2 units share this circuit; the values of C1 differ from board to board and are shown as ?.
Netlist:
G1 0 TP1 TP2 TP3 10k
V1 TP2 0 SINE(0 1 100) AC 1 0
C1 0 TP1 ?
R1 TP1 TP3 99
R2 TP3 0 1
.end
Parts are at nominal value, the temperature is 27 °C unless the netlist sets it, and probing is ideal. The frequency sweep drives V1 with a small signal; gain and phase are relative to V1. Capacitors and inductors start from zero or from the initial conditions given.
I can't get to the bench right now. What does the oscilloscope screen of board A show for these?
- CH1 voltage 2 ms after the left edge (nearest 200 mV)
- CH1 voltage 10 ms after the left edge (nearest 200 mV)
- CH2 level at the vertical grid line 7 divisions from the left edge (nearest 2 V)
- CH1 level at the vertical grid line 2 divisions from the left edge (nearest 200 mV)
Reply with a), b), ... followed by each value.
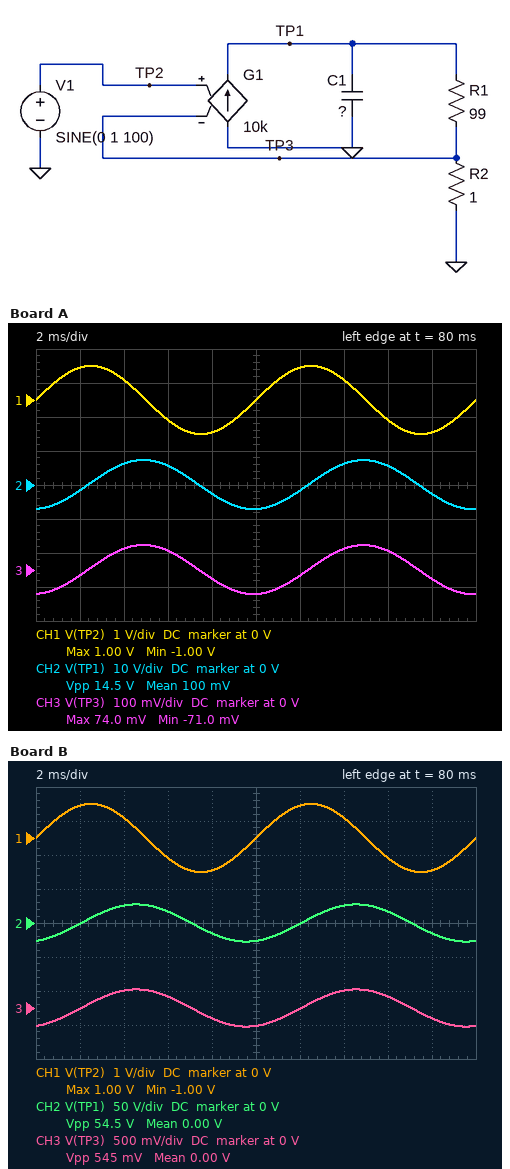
a) 1.0 V
b) 0 V
c) 6 V
d) 600 mV
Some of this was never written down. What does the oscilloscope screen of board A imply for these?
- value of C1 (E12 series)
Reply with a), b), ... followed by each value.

a) 2.2 F
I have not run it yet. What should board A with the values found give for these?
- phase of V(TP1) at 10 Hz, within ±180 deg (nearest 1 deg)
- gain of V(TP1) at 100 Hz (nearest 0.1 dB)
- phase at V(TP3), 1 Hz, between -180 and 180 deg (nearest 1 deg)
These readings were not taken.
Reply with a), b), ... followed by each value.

a) -54 deg
b) 17.2 dB
c) -8 deg
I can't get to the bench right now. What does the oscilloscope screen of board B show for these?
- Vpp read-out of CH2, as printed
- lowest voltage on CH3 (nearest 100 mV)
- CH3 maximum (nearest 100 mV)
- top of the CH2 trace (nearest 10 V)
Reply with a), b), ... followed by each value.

a) 54.5 V
b) -300 mV
c) 300 mV
d) 30 V
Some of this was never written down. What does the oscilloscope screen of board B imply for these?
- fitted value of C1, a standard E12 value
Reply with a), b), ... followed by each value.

a) 560 mF
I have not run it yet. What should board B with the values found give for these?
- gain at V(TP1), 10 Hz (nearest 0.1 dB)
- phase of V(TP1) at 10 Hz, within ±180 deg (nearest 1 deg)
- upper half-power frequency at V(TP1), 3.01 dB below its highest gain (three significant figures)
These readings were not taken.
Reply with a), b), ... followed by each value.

a) 39.5 dB
b) -19 deg
c) 28.4 Hz
